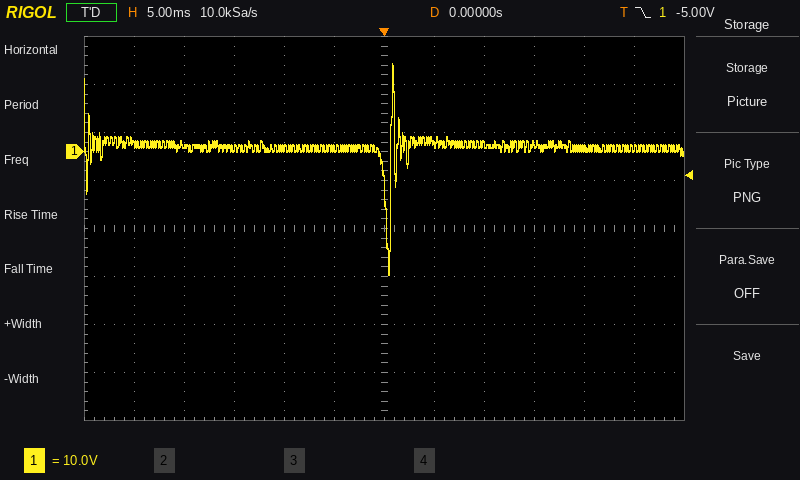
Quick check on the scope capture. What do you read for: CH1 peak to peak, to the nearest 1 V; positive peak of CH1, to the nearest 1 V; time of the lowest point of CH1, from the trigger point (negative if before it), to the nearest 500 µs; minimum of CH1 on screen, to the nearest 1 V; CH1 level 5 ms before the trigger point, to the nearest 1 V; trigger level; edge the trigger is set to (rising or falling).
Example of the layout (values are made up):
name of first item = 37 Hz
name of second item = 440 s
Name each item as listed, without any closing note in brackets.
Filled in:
CH1 peak to peak, to the nearest 1 V = 44 V
positive peak of CH1, to the nearest 1 V = 18 V
time of the lowest point of CH1, from the trigger point (negative if before it), to the nearest 500 µs = +500 µs
minimum of CH1 on screen, to the nearest 1 V = -26 V
CH1 level 5 ms before the trigger point, to the nearest 1 V = 1 V
trigger level = -5.00 V
edge the trigger is set to = falling
